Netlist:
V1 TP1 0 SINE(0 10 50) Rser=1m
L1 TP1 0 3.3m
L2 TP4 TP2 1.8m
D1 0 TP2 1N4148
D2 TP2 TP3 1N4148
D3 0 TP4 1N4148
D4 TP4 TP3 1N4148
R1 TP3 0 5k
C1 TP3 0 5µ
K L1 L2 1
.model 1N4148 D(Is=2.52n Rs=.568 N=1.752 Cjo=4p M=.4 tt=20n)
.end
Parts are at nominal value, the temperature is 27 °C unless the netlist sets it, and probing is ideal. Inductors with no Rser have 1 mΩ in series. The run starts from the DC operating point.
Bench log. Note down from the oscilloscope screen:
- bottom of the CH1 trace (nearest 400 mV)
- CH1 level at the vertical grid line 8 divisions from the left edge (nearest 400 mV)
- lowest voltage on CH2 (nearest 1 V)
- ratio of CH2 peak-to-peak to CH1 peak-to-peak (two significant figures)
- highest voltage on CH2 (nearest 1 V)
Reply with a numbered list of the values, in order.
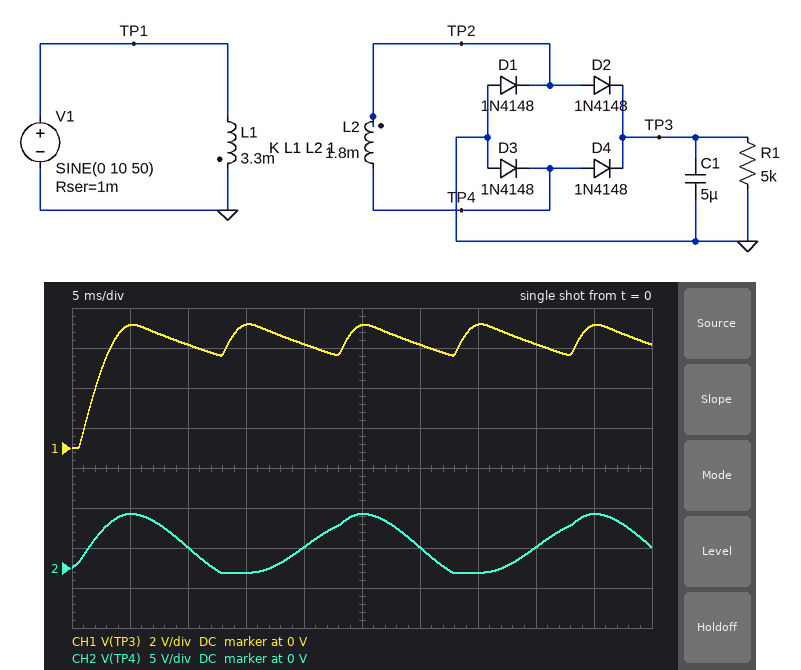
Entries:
1. 0 V
2. 5.2 V
3. -1 V
4. 1.2
5. 7 V
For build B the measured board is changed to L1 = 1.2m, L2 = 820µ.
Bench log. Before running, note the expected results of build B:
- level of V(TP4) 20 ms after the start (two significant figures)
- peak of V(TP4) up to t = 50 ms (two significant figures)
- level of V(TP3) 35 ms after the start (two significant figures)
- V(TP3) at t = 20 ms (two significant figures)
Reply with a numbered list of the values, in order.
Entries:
1. 3.0 V
2. 7.6 V
3. 7.1 V
4. 5.9 V
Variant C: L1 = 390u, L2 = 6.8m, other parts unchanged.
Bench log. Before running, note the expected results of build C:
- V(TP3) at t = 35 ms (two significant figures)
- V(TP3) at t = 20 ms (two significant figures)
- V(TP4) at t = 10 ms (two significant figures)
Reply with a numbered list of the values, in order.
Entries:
1. 41 V
2. 34 V
3. 16 V
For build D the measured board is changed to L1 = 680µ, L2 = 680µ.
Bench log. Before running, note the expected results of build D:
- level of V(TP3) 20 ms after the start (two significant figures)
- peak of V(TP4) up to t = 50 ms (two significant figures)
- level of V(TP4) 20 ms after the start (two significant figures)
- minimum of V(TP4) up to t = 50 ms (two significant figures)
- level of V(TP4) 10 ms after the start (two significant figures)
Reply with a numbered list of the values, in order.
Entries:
1. 7.4 V
2. 9.3 V
3. 3.7 V
4. -700 mV
5. 3.5 V
